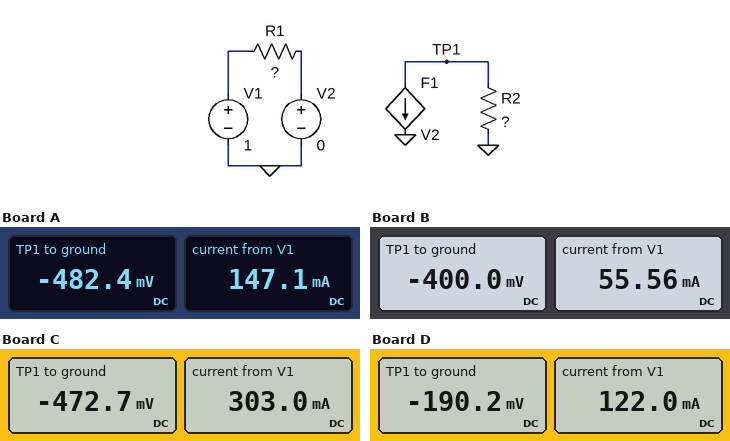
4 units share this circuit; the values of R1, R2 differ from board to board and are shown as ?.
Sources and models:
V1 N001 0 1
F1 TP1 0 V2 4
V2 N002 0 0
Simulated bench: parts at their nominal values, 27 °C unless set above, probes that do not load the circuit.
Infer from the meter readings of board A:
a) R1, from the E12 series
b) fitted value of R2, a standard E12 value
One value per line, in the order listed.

6.8 Ω
0.82 Ω
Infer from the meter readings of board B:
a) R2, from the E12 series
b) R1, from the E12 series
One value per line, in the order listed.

1.8 Ω
18 Ω
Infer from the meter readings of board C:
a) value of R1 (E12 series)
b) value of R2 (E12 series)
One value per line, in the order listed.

3.3 Ω
0.39 Ω
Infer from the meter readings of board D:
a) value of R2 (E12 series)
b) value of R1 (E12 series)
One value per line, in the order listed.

0.39 Ω
8.2 Ω
